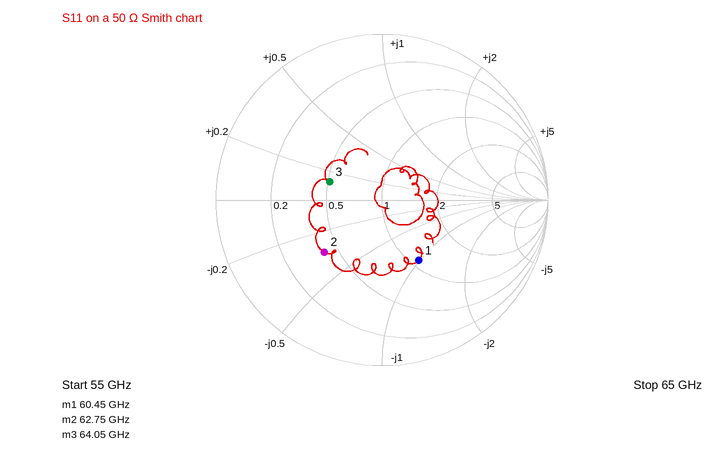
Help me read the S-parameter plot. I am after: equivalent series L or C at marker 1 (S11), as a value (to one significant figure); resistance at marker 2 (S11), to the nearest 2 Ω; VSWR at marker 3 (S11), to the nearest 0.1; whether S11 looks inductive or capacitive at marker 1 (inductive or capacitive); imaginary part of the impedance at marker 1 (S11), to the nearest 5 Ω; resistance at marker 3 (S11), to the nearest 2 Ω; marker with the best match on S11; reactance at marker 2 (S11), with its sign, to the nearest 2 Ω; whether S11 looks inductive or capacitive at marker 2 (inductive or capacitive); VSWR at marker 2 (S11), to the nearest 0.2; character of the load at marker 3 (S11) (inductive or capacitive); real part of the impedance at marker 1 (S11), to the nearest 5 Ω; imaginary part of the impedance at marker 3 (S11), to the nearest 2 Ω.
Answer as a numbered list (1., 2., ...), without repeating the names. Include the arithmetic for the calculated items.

1. C = 1/(2π × 60.45 GHz × 50 Ω) ≈ 52.7 fF, so 50 fF to one significant figure
2. 20 Ω
3. 2.0
4. capacitive
5. -50 Ω
6. 26 Ω
7. marker 3
8. -16 Ω
9. capacitive
10. 2.8
11. inductive
12. 55 Ω
13. +6 Ω
